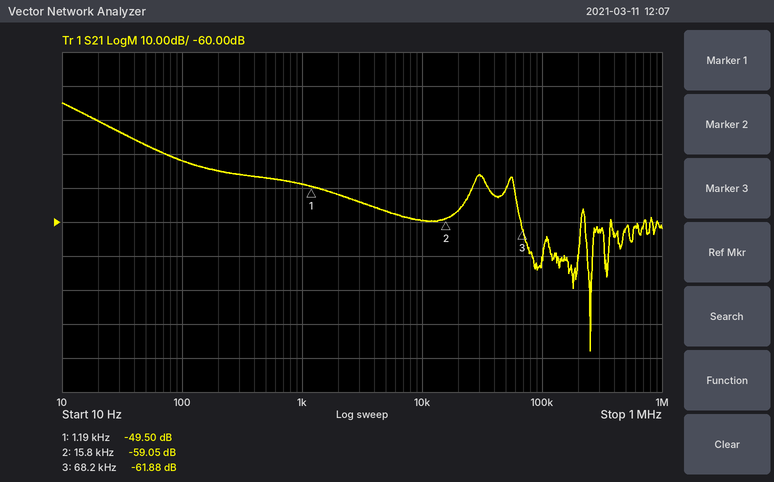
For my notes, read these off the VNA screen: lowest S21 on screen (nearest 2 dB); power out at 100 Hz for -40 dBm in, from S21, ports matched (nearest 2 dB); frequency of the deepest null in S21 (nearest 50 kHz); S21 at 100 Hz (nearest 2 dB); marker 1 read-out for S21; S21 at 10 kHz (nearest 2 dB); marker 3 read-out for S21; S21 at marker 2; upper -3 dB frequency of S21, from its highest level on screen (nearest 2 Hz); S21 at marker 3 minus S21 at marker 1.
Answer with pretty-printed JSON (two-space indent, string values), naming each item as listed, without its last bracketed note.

{
  "lowest S21 on screen": "-98 dB",
  "power out at 100 Hz for -40 dBm in, from S21, ports matched": "-82 dBm",
  "frequency of the deepest null in S21": "250 kHz",
  "S21 at 100 Hz": "-42 dB",
  "marker 1 read-out for S21": "-49.50 dB",
  "S21 at 10 kHz": "-60 dB",
  "marker 3 read-out for S21": "-61.88 dB",
  "S21 at marker 2": "-59.05 dB",
  "upper -3 dB frequency of S21, from its highest level on screen": "14 Hz",
  "S21 at marker 3 minus S21 at marker 1": "-12.38 dB"
}
